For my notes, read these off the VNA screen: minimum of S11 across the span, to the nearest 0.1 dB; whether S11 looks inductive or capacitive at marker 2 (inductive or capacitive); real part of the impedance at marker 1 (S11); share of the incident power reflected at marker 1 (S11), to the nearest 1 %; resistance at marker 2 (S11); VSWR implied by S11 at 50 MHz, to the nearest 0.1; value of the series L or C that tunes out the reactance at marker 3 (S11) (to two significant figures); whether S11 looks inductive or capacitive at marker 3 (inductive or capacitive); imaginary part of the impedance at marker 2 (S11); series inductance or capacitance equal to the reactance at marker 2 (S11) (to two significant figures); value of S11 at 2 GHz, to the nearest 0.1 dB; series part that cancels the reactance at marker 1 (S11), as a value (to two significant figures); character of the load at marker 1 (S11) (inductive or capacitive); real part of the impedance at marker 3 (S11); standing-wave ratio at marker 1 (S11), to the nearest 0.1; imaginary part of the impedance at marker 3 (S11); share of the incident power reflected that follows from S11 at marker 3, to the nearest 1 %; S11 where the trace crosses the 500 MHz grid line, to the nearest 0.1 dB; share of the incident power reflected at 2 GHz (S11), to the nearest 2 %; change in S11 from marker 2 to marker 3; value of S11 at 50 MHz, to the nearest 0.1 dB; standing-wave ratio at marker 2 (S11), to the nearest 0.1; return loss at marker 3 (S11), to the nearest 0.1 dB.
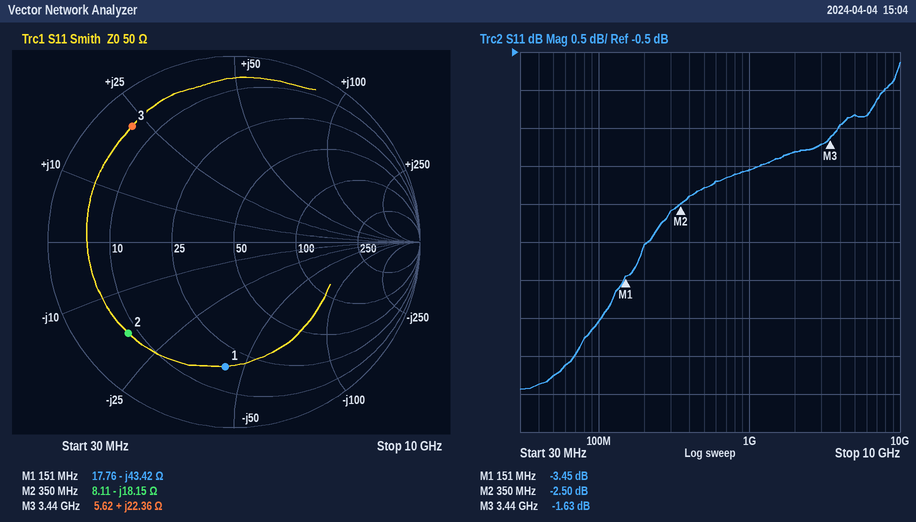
-4.9 dB
capacitive
17.76 Ω
45 %
8.11 Ω
3.7
2.1 pF
inductive
-18.15 Ω
25 pF
-1.8 dB
46 nH
capacitive
5.62 Ω
5.1
+22.36 Ω
69 %
-2.3 dB
66 %
0.87 dB
-4.8 dB
7.0
1.6 dB
